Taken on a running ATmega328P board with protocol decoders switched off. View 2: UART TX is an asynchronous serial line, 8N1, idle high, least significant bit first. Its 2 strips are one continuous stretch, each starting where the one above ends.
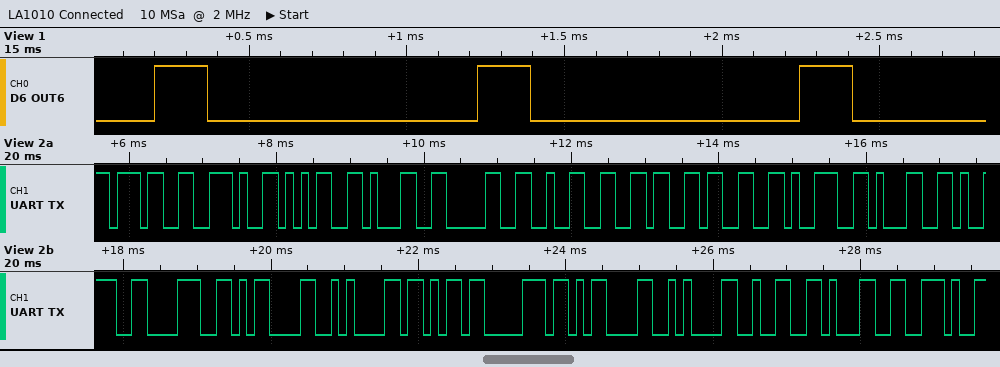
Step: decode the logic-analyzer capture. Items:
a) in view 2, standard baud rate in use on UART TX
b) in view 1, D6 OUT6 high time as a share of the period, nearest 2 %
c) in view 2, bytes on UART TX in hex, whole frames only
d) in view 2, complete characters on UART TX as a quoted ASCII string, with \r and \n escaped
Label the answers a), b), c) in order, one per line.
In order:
a) 9600 baud
b) 16 %
c) 0x37 0x2E 0x35 0x31 0x30 0x32 0x36 0x33 0x39 0x31 0x39 0x38 0x0D 0x0A 0x6B 0x70 0x0D 0x0A 0x32 0x31 0x2E
d) "7.5102639198\r\nkp\r\n21."
